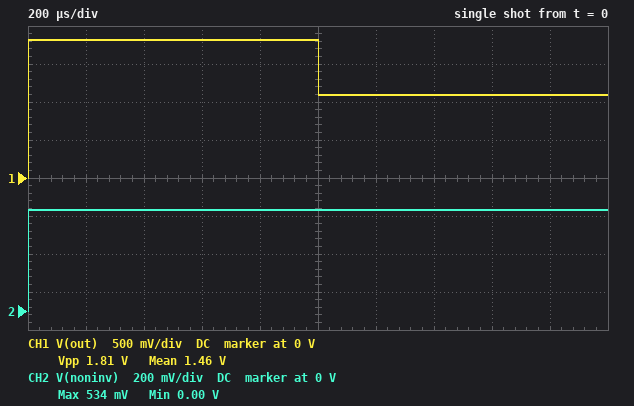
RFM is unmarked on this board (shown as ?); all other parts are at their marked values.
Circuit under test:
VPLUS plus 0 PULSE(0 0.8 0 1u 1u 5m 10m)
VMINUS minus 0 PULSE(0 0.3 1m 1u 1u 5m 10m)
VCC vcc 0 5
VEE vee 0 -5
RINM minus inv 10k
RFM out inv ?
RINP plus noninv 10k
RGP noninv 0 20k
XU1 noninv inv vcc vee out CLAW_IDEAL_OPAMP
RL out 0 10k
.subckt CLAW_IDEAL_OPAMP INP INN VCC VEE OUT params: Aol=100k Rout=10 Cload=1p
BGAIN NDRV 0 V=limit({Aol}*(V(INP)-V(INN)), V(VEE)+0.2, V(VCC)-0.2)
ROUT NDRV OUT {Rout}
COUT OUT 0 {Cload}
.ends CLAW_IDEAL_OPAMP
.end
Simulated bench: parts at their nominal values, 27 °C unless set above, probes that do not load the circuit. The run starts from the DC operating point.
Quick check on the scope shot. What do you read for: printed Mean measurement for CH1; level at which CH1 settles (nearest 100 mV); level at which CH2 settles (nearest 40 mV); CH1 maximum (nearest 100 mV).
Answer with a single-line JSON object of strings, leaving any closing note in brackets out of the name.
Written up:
{"printed Mean measurement for CH1": "1.46 V", "level at which CH1 settles": "1.1 V", "level at which CH2 settles": "520 mV", "CH1 maximum": "1.8 V"}
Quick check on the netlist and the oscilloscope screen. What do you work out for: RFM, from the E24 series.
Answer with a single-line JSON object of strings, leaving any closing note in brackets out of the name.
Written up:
{"RFM, from the E24 series": "24 kΩ"}
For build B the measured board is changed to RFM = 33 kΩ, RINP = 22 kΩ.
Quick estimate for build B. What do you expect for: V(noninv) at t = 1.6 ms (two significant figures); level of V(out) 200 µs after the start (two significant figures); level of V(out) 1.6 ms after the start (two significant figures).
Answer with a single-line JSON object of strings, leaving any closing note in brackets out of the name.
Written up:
{"V(noninv) at t = 1.6 ms": "380 mV", "level of V(out) 200 µs after the start": "1.6 V", "level of V(out) 1.6 ms after the start": "650 mV"}
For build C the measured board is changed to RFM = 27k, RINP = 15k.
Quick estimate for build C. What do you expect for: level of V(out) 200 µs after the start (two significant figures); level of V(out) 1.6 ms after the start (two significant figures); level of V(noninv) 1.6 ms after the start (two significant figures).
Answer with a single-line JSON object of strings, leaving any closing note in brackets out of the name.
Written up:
{"level of V(out) 200 µs after the start": "1.7 V", "level of V(out) 1.6 ms after the start": "880 mV", "level of V(noninv) 1.6 ms after the start": "460 mV"}
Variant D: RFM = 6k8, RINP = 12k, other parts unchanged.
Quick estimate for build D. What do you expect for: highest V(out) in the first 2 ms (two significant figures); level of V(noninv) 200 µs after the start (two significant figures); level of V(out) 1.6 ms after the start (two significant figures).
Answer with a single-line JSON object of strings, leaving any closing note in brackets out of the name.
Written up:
{"highest V(out) in the first 2 ms": "840 mV", "level of V(noninv) 200 µs after the start": "500 mV", "level of V(out) 1.6 ms after the start": "640 mV"}
